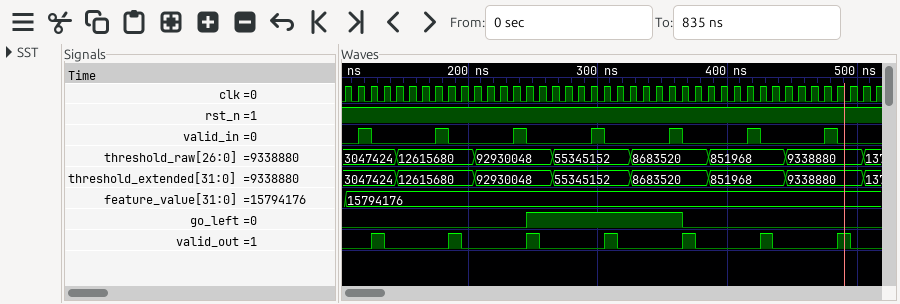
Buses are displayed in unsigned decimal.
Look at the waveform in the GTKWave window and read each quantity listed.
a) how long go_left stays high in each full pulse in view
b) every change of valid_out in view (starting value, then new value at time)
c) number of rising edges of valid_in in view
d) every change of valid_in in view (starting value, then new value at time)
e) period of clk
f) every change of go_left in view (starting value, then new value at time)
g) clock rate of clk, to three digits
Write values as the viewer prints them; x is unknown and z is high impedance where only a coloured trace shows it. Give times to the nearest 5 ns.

120 ns
0, 1 at 125 ns, 0 at 135 ns, 1 at 185 ns, 0 at 195 ns, 1 at 245 ns, 0 at 255 ns, 1 at 305 ns, 0 at 315 ns, 1 at 365 ns, 0 at 375 ns, 1 at 425 ns, 0 at 435 ns, 1 at 485 ns, 0 at 495 ns
7
0, 1 at 115 ns, 0 at 125 ns, 1 at 175 ns, 0 at 185 ns, 1 at 235 ns, 0 at 245 ns, 1 at 295 ns, 0 at 305 ns, 1 at 355 ns, 0 at 365 ns, 1 at 415 ns, 0 at 425 ns, 1 at 475 ns, 0 at 485 ns
10 ns
0, 1 at 245 ns, 0 at 365 ns
100 MHz
